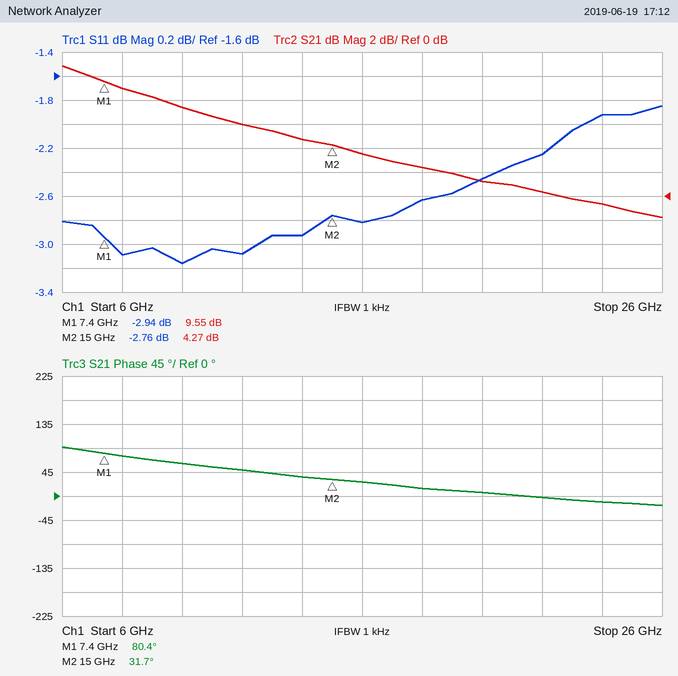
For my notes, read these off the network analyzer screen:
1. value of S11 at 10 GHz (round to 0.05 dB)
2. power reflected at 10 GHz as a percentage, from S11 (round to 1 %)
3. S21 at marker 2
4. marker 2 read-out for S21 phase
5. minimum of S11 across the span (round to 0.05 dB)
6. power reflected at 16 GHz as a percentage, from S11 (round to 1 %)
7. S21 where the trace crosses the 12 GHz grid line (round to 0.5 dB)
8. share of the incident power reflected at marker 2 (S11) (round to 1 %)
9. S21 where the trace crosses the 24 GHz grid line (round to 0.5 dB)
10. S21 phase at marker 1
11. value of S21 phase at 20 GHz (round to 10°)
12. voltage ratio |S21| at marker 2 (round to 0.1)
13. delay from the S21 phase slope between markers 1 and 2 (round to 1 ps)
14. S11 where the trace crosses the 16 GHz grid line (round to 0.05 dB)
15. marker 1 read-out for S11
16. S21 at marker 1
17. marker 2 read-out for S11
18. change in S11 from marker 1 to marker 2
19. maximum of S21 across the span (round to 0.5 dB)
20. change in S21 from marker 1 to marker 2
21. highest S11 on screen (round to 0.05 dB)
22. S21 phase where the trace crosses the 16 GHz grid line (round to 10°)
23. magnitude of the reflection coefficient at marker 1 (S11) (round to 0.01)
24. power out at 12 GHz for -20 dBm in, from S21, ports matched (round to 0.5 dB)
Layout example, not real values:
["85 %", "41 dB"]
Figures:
["-3.15 dB", "48 %", "4.27 dB", "31.7°", "-3.15 dB", "52 %", "6.0 dB", "53 %", "-0.5 dB", "80.4°", "10°", "1.6", "18 ps", "-2.80 dB", "-2.94 dB", "9.55 dB", "-2.76 dB", "0.18 dB", "11.0 dB", "-5.28 dB", "-1.85 dB", "30°", "0.71", "-14.0 dBm"]
